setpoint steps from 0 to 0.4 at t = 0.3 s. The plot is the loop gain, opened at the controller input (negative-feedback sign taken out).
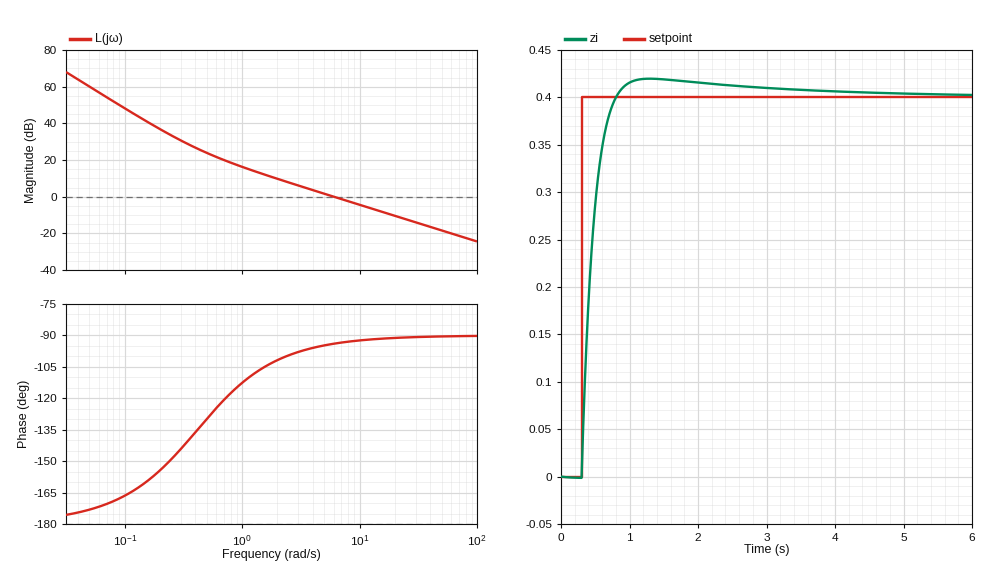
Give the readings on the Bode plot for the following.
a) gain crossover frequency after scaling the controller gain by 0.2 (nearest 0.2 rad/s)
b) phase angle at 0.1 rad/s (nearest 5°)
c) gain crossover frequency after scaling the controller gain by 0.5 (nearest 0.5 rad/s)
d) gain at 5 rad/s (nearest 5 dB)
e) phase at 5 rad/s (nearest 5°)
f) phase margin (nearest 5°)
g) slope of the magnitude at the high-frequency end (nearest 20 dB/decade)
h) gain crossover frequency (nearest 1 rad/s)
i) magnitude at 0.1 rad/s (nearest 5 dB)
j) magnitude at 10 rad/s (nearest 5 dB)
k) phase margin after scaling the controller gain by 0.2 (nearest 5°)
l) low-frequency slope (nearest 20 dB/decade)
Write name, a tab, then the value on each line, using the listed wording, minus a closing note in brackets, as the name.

gain crossover frequency after scaling the controller gain by 0.2	1.2 rad/s
phase angle at 0.1 rad/s	-165°
gain crossover frequency after scaling the controller gain by 0.5	3.0 rad/s
gain at 5 rad/s	0 dB
phase at 5 rad/s	-95°
phase margin	85°
slope of the magnitude at the high-frequency end	-20 dB/decade
gain crossover frequency	6 rad/s
magnitude at 0.1 rad/s	50 dB
magnitude at 10 rad/s	-5 dB
phase margin after scaling the controller gain by 0.2	70°
low-frequency slope	-40 dB/decade
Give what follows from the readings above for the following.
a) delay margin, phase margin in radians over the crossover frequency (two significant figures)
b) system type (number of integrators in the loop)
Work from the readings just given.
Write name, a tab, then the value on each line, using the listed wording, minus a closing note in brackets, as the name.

delay margin, phase margin in radians over the crossover frequency	0.25 s
system type	2
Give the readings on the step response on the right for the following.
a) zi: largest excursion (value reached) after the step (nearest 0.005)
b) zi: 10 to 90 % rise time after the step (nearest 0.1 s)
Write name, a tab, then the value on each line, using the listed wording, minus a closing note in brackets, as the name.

zi: largest excursion (value reached) after the step	0.420
zi: 10 to 90 % rise time after the step	0.3 s
